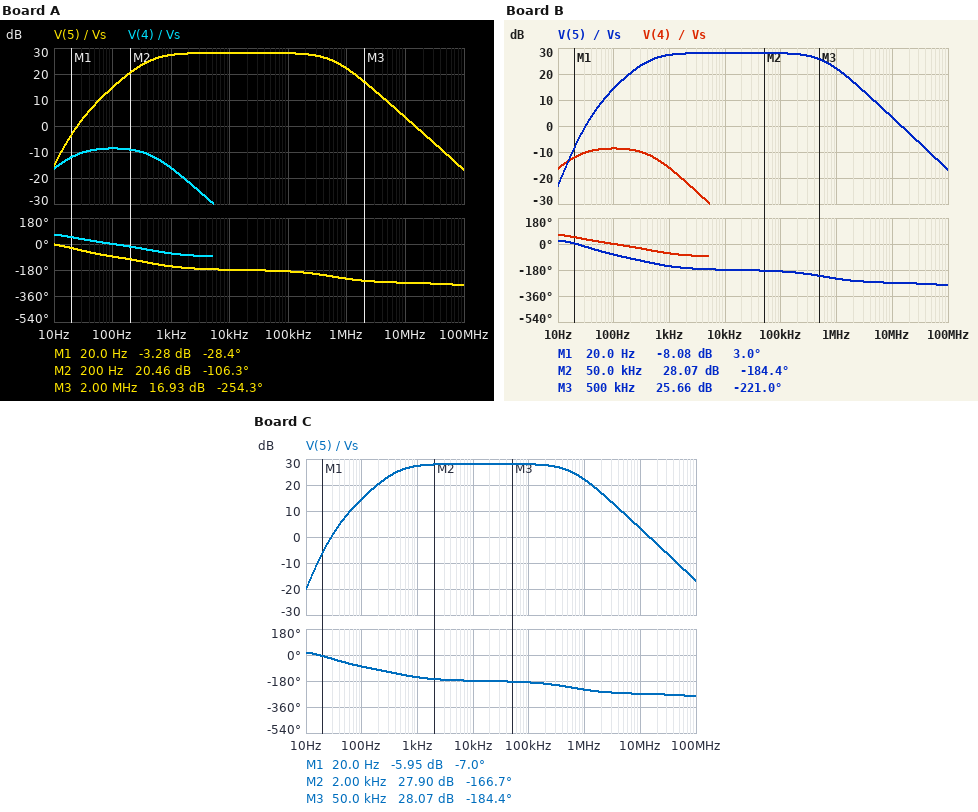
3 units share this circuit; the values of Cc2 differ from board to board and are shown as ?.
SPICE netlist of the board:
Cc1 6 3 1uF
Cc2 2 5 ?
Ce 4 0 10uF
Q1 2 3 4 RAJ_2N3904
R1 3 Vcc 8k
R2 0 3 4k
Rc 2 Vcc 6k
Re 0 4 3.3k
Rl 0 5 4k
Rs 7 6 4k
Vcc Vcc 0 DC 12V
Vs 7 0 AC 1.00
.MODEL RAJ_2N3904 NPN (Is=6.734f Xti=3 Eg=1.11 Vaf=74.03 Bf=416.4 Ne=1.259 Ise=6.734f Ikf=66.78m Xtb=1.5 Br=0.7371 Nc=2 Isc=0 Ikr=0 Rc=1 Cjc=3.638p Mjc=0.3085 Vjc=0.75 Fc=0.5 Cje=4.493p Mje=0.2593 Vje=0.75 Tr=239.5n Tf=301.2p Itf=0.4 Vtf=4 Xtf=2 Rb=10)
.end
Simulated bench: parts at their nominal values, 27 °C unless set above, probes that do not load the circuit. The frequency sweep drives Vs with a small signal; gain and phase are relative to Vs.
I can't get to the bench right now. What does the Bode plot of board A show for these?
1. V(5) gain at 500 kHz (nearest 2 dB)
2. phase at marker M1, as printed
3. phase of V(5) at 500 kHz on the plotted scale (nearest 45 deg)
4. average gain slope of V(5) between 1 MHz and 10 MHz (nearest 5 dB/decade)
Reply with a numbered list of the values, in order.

1. 26 dB
2. -28.4 deg
3. -225 deg
4. -20 dB/decade
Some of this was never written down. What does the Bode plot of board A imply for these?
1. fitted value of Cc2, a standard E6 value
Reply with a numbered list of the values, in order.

1. 1.5 µF
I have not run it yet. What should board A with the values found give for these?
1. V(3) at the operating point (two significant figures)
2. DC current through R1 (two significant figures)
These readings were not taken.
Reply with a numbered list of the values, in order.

1. 4.0 V
2. 1.0 mA
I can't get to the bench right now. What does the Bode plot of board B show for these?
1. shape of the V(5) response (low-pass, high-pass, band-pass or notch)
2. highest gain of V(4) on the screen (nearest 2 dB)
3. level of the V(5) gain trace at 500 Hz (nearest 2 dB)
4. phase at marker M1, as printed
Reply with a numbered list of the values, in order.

1. band-pass
2. -8 dB
3. 26 dB
4. 3.0 deg
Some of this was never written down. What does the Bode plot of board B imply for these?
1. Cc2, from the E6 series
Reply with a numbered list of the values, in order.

1. 470 nF
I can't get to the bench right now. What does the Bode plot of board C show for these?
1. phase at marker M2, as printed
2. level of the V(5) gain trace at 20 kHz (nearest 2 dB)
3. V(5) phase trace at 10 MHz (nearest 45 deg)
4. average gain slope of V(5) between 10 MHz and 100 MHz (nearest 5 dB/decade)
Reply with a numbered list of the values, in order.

1. -166.7 deg
2. 28 dB
3. -270 deg
4. -20 dB/decade
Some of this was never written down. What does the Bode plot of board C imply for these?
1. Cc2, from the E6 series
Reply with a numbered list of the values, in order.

1. 680 nF
